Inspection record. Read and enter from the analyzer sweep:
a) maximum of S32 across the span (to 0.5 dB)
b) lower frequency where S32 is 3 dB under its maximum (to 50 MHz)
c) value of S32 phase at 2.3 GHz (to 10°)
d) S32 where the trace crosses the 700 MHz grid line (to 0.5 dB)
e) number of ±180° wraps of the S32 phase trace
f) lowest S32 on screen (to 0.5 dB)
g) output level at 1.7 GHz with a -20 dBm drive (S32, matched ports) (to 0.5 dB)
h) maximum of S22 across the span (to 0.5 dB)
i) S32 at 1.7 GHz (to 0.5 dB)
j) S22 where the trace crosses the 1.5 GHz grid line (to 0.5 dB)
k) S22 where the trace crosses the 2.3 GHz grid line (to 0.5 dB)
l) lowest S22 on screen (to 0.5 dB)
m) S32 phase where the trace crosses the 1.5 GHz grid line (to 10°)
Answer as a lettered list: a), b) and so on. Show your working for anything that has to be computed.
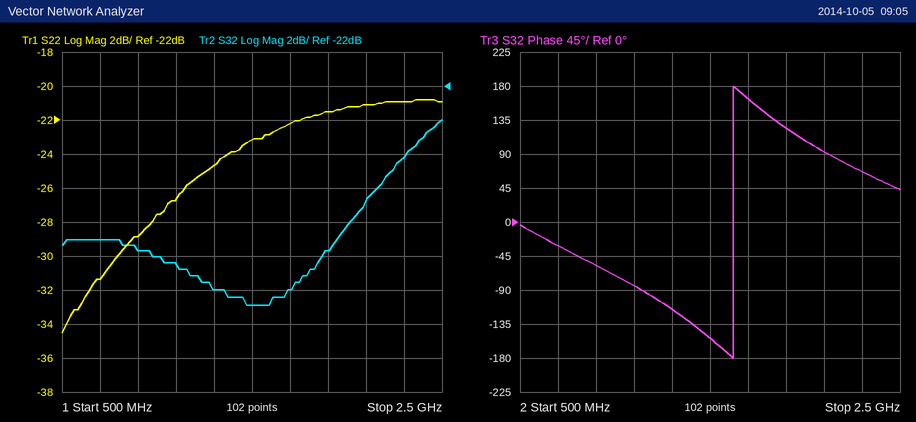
a) -24.0 dB
b) 2.25 GHz
c) 70°
d) -31.0 dB
e) 1
f) -35.0 dB
g) -20 dBm + (-34.0 dB) = -54.0 dBm
h) -21.0 dB
i) -34.0 dB
j) -23.0 dB
k) -21.0 dB
l) -34.5 dB
m) -150°
